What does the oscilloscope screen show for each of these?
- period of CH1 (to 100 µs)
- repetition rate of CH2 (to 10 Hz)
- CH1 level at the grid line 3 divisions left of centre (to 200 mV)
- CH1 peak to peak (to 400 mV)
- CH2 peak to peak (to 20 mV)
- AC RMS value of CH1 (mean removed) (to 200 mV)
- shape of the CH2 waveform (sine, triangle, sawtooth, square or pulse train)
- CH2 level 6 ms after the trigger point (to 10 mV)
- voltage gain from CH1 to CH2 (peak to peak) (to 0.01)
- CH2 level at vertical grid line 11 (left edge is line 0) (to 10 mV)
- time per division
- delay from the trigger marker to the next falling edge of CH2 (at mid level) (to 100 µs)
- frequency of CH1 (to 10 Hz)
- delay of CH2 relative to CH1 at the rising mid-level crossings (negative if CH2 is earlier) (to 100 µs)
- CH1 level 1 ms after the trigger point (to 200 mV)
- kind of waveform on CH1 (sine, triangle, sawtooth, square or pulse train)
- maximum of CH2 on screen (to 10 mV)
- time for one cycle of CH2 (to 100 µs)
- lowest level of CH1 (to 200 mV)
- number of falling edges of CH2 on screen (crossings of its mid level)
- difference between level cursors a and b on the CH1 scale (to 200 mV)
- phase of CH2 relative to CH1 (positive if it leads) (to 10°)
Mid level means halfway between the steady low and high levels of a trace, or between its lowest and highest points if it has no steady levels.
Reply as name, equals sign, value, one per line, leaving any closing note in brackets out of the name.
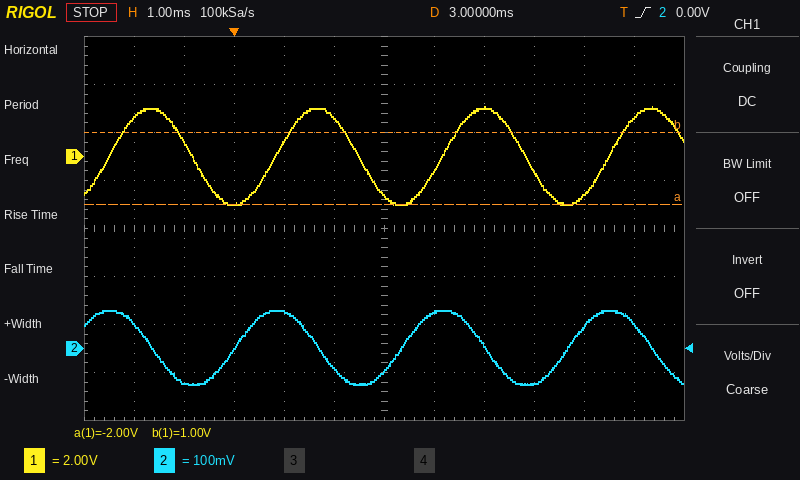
period of CH1 = 3.3 ms
repetition rate of CH2 = 300 Hz
CH1 level at the grid line 3 divisions left of centre = -2.0 V
CH1 peak to peak = 4.0 V
CH2 peak to peak = 160 mV
AC RMS value of CH1 (mean removed) = 1.4 V
shape of the CH2 waveform = sine
CH2 level 6 ms after the trigger point = -70 mV
voltage gain from CH1 to CH2 (peak to peak) = 0.04
CH2 level at vertical grid line 11 (left edge is line 0) = 50 mV
time per division = 1 ms
delay from the trigger marker to the next falling edge of CH2 (at mid level) = 1.7 ms
frequency of CH1 = 300 Hz
delay of CH2 relative to CH1 at the rising mid-level crossings (negative if CH2 is earlier) = -800 µs
CH1 level 1 ms after the trigger point = 600 mV
kind of waveform on CH1 = sine
maximum of CH2 on screen = 80 mV
time for one cycle of CH2 = 3.3 ms
lowest level of CH1 = -2.0 V
number of falling edges of CH2 on screen = 4
difference between level cursors a and b on the CH1 scale = 3.0 V
phase of CH2 relative to CH1 (positive if it leads) = +90°
